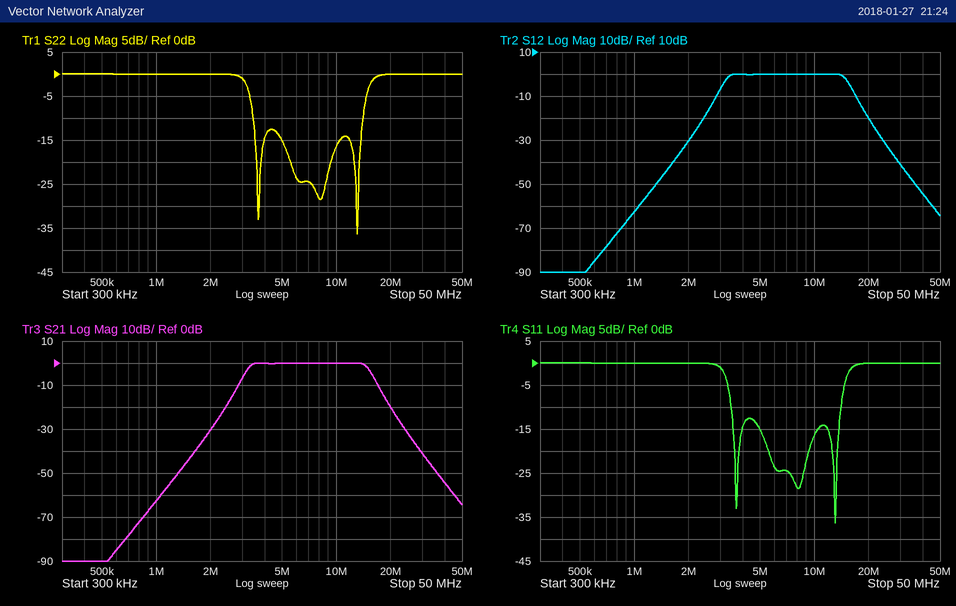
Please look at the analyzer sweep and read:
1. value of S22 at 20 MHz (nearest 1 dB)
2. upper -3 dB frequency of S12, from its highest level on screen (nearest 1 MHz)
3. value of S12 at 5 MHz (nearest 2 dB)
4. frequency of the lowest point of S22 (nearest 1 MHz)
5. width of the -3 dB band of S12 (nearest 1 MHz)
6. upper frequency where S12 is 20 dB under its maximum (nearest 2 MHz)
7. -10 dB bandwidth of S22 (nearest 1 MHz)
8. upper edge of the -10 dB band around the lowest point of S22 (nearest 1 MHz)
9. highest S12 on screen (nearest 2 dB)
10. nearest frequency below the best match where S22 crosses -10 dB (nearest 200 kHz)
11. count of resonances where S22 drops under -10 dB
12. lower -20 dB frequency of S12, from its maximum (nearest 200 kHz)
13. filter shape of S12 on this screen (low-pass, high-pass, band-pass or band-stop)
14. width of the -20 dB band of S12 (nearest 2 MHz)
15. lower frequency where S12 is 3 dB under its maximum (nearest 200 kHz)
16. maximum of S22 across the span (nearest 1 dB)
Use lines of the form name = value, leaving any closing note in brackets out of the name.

value of S22 at 20 MHz = 0 dB
upper -3 dB frequency of S12, from its highest level on screen = 15 MHz
value of S12 at 5 MHz = 0 dB
frequency of the lowest point of S22 = 13 MHz
width of the -3 dB band of S12 = 12 MHz
upper frequency where S12 is 20 dB under its maximum = 20 MHz
-10 dB bandwidth of S22 = 11 MHz
upper edge of the -10 dB band around the lowest point of S22 = 14 MHz
highest S12 on screen = 0 dB
nearest frequency below the best match where S22 crosses -10 dB = 3.4 MHz
count of resonances where S22 drops under -10 dB = 3
lower -20 dB frequency of S12, from its maximum = 2.4 MHz
filter shape of S12 on this screen = band-pass
width of the -20 dB band of S12 = 18 MHz
lower frequency where S12 is 3 dB under its maximum = 3.2 MHz
maximum of S22 across the span = 0 dB
